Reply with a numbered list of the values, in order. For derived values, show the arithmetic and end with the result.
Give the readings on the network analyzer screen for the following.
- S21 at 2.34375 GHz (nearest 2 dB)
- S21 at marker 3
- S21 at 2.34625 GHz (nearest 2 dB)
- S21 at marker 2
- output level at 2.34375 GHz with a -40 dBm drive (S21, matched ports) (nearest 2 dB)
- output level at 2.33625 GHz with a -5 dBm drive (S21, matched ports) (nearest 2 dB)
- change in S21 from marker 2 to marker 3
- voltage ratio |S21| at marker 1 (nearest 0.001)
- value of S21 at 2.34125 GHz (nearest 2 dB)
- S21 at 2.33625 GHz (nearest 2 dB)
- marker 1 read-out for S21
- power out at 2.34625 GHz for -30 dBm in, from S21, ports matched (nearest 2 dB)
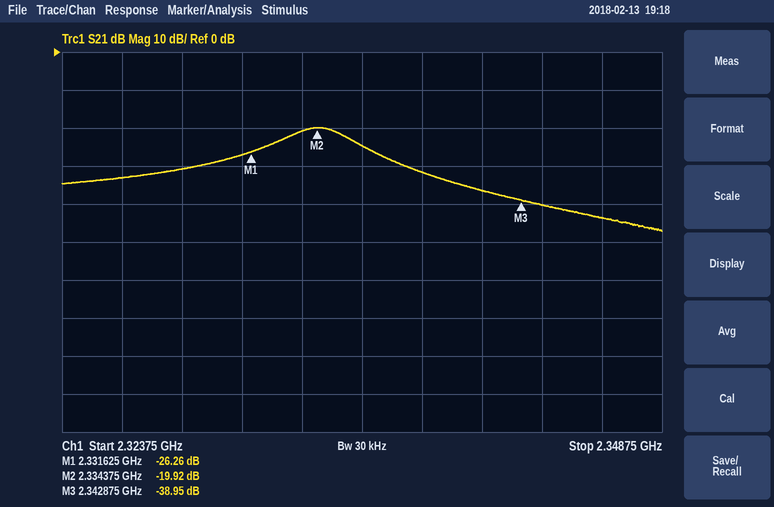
1. -40 dB
2. -38.95 dB
3. -44 dB
4. -19.92 dB
5. -40 dBm + (-40 dB) = -80 dBm
6. -5 dBm + (-24 dB) = -30 dBm
7. -38.95 − (-19.92) = -19.03 dB
8. 10^(-26.26/20) ≈ 0.049
9. -36 dB
10. -24 dB
11. -26.26 dB
12. -30 dBm + (-44 dB) = -74 dBm
